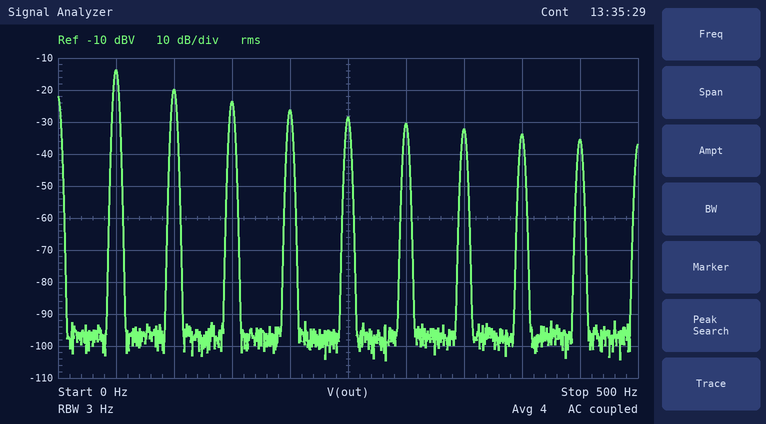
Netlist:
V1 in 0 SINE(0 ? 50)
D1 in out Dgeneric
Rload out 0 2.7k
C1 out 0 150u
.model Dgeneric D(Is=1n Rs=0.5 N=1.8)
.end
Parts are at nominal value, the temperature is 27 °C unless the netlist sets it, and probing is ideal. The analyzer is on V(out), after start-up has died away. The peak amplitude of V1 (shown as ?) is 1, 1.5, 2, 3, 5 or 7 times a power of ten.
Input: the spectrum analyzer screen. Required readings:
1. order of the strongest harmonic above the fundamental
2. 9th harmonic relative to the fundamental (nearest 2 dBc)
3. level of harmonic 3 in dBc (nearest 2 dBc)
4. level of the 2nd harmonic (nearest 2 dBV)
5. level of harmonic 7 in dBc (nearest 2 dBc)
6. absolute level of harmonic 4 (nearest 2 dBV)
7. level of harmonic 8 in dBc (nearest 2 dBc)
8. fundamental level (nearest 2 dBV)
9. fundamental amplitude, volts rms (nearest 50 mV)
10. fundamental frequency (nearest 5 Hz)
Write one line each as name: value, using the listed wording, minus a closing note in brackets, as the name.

order of the strongest harmonic above the fundamental: 2
9th harmonic relative to the fundamental: -22 dBc
level of harmonic 3 in dBc: -10 dBc
level of the 2nd harmonic: -20 dBV
level of harmonic 7 in dBc: -18 dBc
absolute level of harmonic 4: -26 dBV
level of harmonic 8 in dBc: -20 dBc
fundamental level: -14 dBV
fundamental amplitude, volts rms: 200 mV
fundamental frequency: 50 Hz
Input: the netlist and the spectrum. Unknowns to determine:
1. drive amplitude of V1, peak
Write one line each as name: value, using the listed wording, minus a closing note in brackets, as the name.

drive amplitude of V1, peak: 20 V
